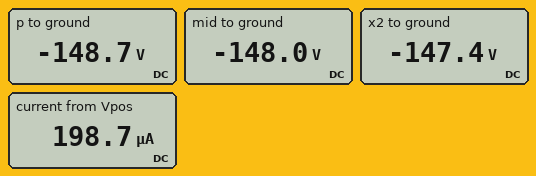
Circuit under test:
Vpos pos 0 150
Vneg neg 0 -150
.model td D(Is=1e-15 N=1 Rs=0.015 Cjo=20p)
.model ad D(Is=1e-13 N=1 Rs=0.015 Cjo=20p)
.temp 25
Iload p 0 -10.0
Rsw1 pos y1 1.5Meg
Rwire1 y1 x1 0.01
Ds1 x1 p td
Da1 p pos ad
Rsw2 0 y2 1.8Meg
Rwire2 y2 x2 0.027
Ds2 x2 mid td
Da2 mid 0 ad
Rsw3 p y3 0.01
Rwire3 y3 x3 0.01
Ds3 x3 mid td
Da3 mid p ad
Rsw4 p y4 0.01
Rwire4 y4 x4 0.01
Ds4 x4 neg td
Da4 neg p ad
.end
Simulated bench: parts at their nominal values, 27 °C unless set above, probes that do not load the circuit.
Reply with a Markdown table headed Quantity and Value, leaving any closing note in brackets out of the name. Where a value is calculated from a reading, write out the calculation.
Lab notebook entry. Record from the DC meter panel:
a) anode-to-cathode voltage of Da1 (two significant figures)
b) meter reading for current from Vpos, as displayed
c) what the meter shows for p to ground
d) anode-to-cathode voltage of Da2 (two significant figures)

| Quantity | Value |
|---|---|
| anode-to-cathode voltage of Da1 | -148.7 V - 150 V = -300 V |
| meter reading for current from Vpos, as displayed | 198.7 µA |
| what the meter shows for p to ground | -148.7 V |
| anode-to-cathode voltage of Da2 | -148 V = -150 V |
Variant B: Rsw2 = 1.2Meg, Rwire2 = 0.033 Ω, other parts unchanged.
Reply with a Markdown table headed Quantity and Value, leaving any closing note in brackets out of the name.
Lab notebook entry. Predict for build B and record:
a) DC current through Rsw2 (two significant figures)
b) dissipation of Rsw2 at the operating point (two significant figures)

| Quantity | Value |
|---|---|
| DC current through Rsw2 | 120 µA |
| dissipation of Rsw2 at the operating point | 18 mW |
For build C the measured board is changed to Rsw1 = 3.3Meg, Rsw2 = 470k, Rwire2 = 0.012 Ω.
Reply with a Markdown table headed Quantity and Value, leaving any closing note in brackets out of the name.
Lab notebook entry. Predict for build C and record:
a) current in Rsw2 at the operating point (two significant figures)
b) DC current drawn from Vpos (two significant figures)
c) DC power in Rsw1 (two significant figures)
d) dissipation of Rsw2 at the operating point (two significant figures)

| Quantity | Value |
|---|---|
| current in Rsw2 at the operating point | 310 µA |
| DC current drawn from Vpos | 90 µA |
| DC power in Rsw1 | 27 mW |
| dissipation of Rsw2 at the operating point | 46 mW |
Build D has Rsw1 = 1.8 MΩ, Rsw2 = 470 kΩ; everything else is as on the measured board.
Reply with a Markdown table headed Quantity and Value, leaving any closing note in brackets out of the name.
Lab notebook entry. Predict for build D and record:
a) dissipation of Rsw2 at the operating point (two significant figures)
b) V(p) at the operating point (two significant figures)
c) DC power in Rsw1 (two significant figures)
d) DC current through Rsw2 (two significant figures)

| Quantity | Value |
|---|---|
| dissipation of Rsw2 at the operating point | 46 mW |
| V(p) at the operating point | -150 V |
| DC power in Rsw1 | 49 mW |
| DC current through Rsw2 | 310 µA |
